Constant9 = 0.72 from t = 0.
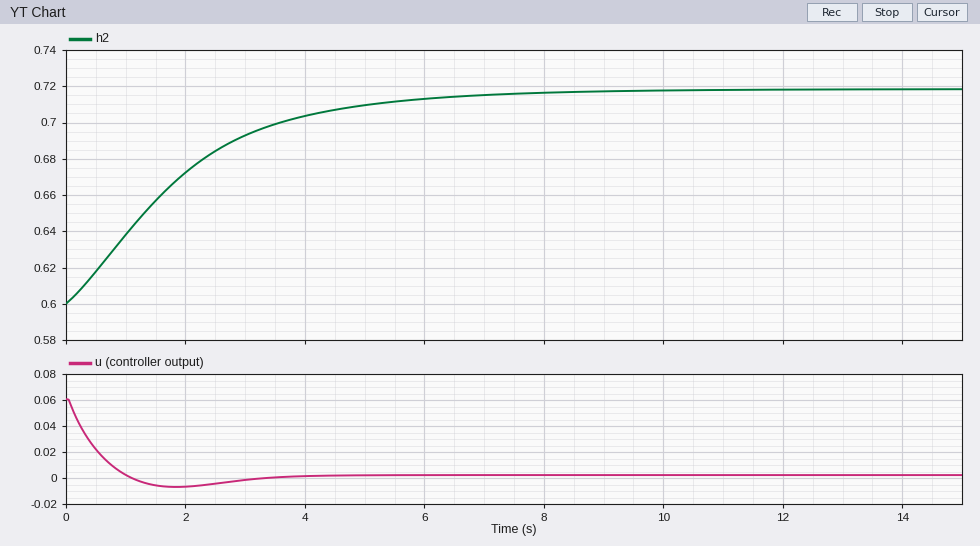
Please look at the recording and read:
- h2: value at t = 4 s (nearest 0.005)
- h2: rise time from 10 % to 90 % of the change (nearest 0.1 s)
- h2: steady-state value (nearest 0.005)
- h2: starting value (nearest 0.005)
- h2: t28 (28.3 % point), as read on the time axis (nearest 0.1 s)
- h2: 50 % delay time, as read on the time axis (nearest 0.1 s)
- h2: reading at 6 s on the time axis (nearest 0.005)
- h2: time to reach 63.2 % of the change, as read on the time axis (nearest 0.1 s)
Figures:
0.705
4.1 s
0.720
0.600
0.9 s
1.6 s
0.715
2.1 s
